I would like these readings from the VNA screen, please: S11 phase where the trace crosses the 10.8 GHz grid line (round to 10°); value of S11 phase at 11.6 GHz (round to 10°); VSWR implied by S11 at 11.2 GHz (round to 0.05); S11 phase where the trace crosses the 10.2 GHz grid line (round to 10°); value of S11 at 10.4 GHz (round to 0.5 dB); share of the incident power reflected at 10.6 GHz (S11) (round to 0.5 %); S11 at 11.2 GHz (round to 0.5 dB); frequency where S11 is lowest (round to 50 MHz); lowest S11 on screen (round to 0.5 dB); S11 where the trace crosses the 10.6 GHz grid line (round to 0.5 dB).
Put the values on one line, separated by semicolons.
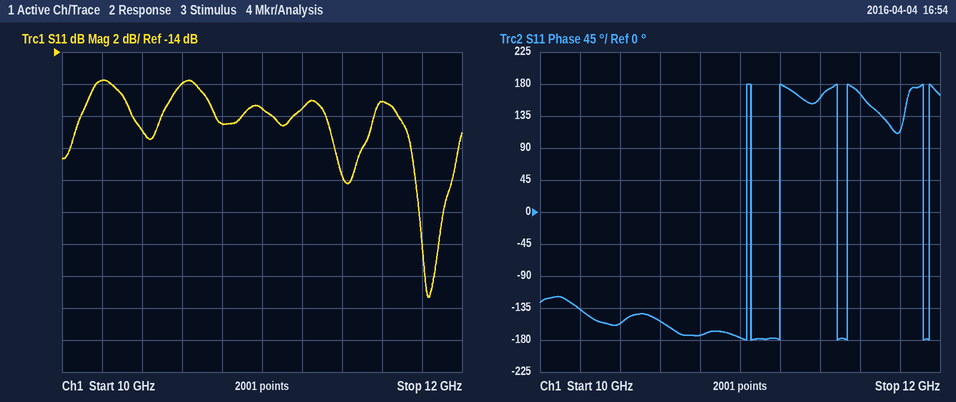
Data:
-170°; 170°; 1.30; -140°; -19.0 dB; 2.5 %; -17.5 dB; 11.85 GHz; -29.5 dB; -16.0 dB
